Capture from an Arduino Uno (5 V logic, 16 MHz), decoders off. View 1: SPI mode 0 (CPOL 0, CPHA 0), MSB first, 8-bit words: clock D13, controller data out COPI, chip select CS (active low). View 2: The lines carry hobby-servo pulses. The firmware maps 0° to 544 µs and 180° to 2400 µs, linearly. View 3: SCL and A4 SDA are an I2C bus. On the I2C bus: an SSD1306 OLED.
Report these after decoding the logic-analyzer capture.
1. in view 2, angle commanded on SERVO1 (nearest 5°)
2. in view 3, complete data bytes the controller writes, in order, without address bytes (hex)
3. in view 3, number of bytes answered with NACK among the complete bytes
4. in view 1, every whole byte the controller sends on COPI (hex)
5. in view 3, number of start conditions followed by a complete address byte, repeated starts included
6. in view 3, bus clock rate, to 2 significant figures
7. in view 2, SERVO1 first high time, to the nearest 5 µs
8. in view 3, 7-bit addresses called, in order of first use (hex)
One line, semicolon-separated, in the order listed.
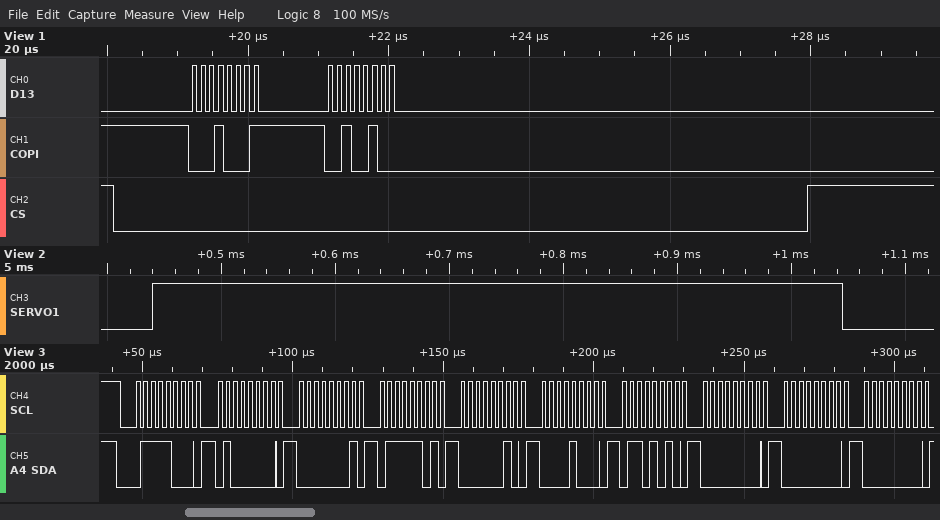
5°; 40 01 7D 02 08 6A 00 00 00; 0; 11 24; 1; 400 kHz; 605 µs; 0x3C
